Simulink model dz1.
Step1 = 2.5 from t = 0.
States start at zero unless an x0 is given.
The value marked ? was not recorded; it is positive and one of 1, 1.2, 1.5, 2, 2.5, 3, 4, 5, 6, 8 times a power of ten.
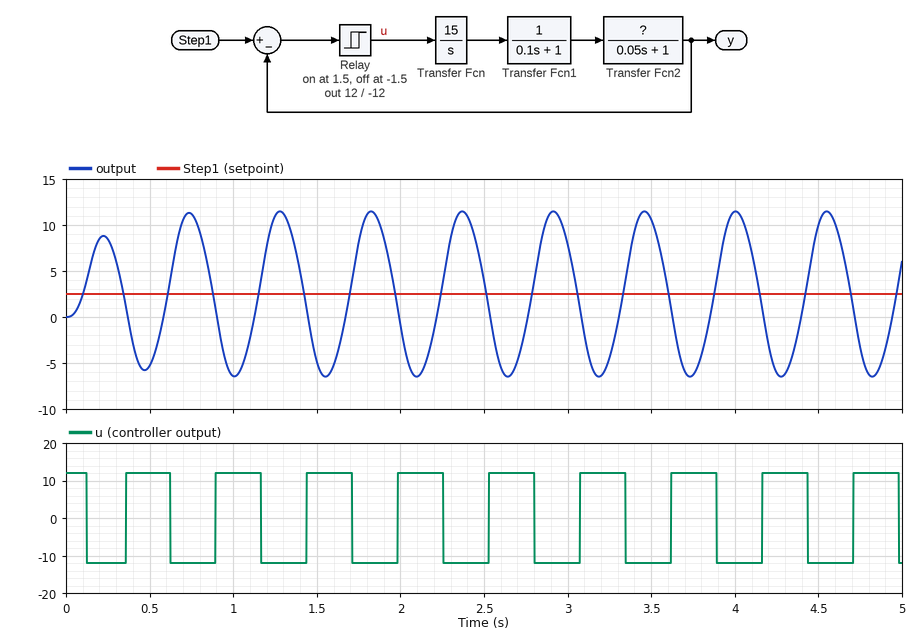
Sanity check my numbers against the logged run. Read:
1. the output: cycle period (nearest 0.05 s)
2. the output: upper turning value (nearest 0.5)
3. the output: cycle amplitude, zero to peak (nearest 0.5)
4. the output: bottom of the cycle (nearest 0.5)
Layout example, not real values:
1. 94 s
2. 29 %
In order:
1. 0.55 s
2. 11.5
3. 9.0
4. -6.5
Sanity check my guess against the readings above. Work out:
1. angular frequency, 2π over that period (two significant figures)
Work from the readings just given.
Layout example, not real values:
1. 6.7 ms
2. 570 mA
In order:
1. 11 rad/s
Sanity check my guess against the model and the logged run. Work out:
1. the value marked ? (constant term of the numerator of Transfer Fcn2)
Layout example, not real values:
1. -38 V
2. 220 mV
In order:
1. 0.8
